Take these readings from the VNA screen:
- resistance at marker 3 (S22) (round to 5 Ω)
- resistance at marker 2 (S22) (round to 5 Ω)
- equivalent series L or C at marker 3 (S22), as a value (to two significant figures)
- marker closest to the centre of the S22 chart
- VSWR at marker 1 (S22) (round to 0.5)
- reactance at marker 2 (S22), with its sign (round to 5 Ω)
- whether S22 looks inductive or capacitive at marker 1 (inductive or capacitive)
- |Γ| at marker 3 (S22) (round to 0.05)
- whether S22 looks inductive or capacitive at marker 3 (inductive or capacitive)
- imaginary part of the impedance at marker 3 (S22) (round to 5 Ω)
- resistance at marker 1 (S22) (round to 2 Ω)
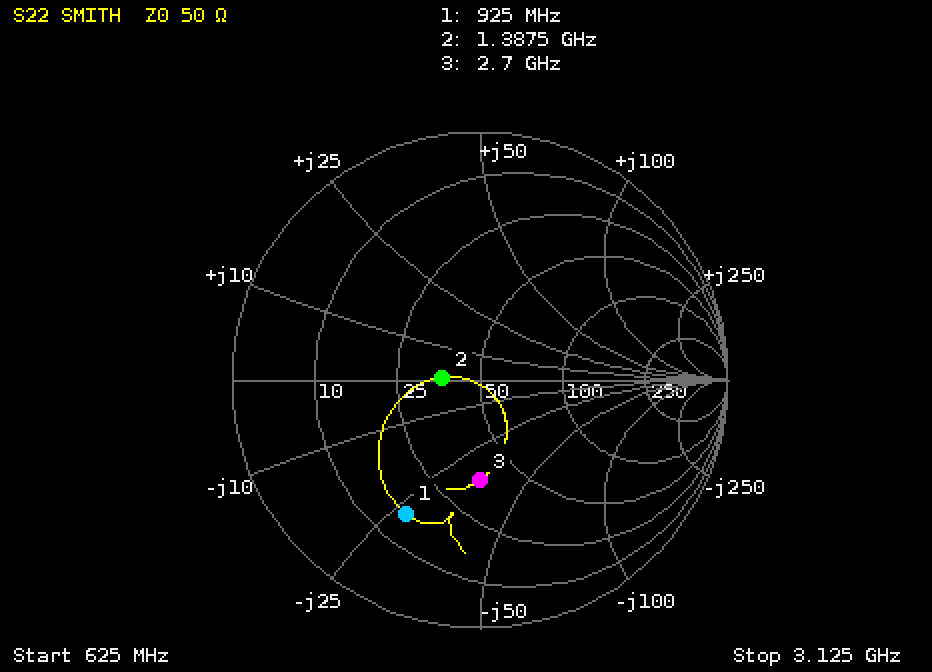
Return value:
35 Ω
35 Ω
1.7 pF
marker 2
4.0
0 Ω
capacitive
0.40
capacitive
-35 Ω
16 Ω
